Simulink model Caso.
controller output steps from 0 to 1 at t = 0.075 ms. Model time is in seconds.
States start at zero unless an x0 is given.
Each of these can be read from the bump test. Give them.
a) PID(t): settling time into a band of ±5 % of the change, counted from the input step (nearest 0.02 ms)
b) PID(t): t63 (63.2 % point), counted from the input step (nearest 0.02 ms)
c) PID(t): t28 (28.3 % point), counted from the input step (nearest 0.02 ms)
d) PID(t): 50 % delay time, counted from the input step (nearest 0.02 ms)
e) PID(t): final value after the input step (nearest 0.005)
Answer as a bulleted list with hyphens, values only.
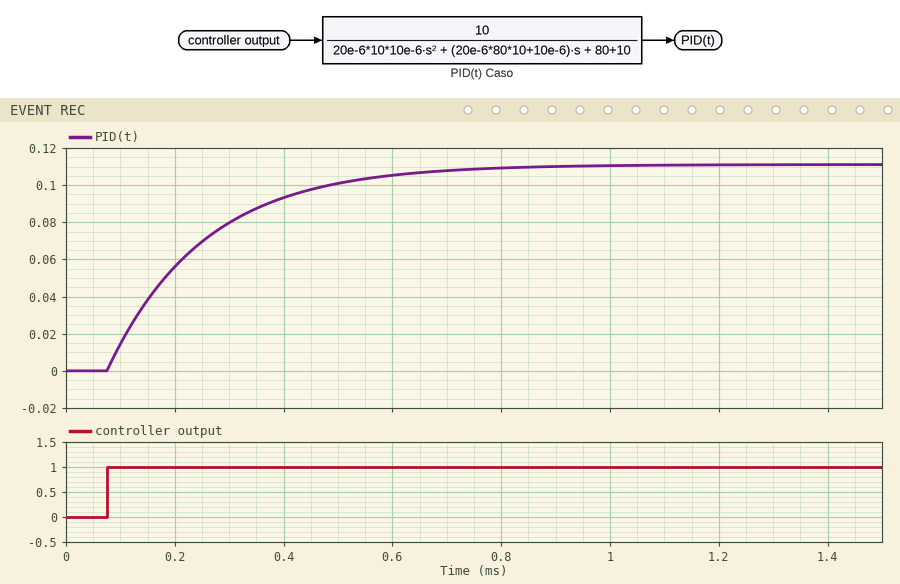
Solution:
- 0.54 ms
- 0.18 ms
- 0.06 ms
- 0.12 ms
- 0.110
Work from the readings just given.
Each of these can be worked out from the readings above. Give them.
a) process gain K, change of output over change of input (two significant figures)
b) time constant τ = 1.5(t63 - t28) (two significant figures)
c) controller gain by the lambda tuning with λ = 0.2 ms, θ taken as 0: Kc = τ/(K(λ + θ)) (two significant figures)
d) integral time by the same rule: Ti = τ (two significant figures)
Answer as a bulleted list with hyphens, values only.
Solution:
- 0.11
- 0.18 ms
- 8.2
- 0.18 ms
